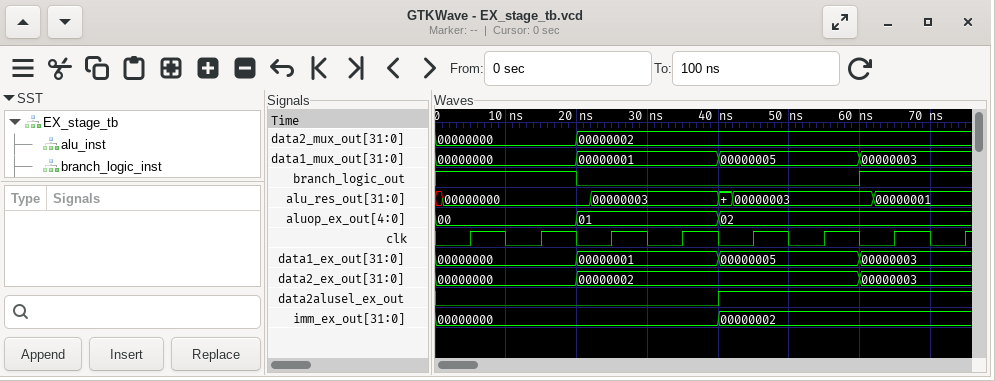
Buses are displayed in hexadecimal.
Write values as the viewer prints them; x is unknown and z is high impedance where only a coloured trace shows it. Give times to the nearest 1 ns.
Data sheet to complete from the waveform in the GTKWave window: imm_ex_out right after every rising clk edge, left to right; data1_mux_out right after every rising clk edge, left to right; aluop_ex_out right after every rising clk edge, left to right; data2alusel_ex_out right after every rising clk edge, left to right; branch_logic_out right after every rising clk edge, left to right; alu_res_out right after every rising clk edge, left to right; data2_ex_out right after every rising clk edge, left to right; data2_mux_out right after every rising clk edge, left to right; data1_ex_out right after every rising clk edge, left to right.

00000000, 00000000, 00000000, 00000000, 00000002, 00000002, 00000002, 00000002
00000000, 00000000, 00000001, 00000001, 00000005, 00000005, 00000003, 00000003
00, 00, 01, 01, 02, 02, 02, 02
0 0 0 0 1 1 1 1
1 1 0 0 0 0 1 1
00000000, 00000000, 00000003, 00000003, 00000003, 00000003, 00000001, 00000001
00000000, 00000000, 00000002, 00000002, 00000002, 00000002, 00000003, 00000003
00000000, 00000000, 00000002, 00000002, 00000002, 00000002, 00000002, 00000002
00000000, 00000000, 00000001, 00000001, 00000005, 00000005, 00000003, 00000003
